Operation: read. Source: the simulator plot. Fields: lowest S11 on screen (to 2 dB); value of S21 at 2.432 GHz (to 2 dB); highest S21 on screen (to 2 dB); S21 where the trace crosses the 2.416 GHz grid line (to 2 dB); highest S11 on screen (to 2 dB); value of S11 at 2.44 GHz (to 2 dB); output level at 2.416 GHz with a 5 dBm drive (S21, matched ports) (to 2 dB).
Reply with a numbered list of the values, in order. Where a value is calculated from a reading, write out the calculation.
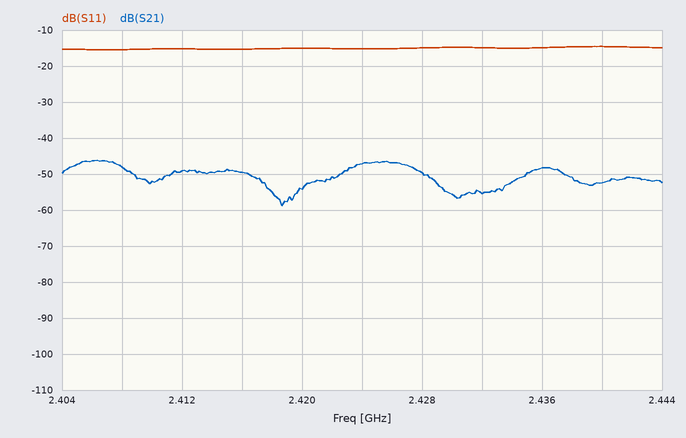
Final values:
1. -16 dB
2. -56 dB
3. -46 dB
4. -50 dB
5. -14 dB
6. -14 dB
7. 5 dBm + (-50 dB) = -44 dBm
